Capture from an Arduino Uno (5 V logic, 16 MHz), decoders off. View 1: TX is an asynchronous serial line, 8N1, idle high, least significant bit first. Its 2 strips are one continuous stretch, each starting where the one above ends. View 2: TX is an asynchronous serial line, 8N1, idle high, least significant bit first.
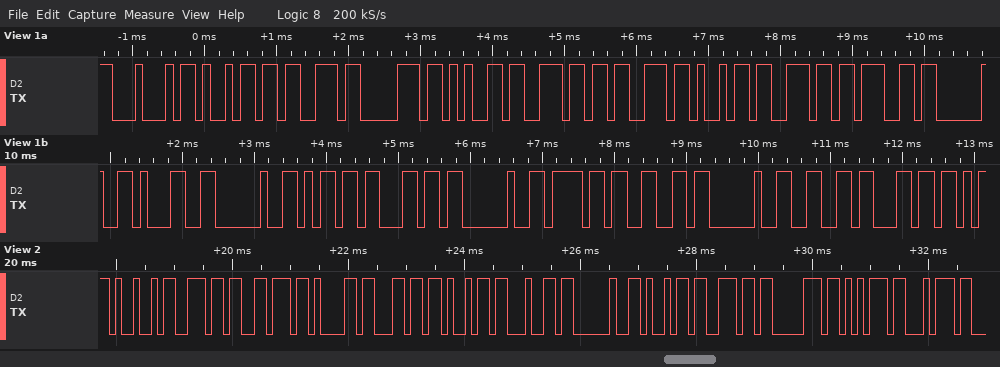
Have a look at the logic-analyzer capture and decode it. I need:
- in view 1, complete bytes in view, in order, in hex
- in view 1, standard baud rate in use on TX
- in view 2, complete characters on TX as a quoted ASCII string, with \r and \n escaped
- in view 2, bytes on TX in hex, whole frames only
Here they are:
44 69 73 70 65 6E 73 69 6E 67 20 31 20 6D 6C 20 6F 66 20 66 6C
9600 baud
"Invalid input"
49 6E 76 61 6C 69 64 20 69 6E 70 75 74
